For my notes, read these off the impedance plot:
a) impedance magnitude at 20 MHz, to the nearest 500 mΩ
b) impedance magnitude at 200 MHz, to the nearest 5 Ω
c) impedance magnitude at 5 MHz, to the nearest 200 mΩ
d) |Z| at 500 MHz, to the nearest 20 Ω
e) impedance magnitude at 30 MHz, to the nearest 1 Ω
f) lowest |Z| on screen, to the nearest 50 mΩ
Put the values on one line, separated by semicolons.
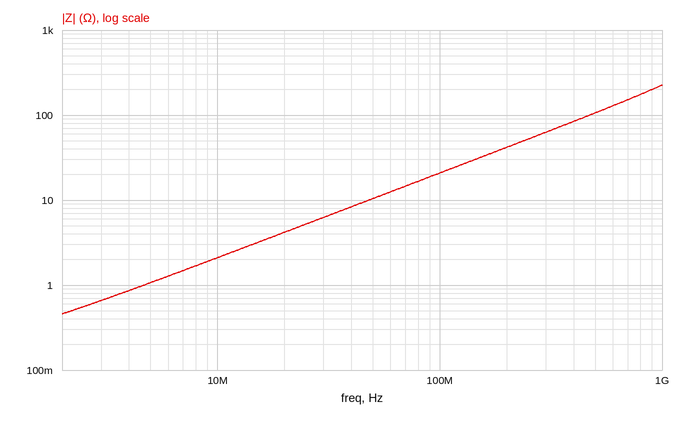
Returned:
4.0 Ω; 40 Ω; 1.0 Ω; 100 Ω; 6 Ω; 450 mΩ
